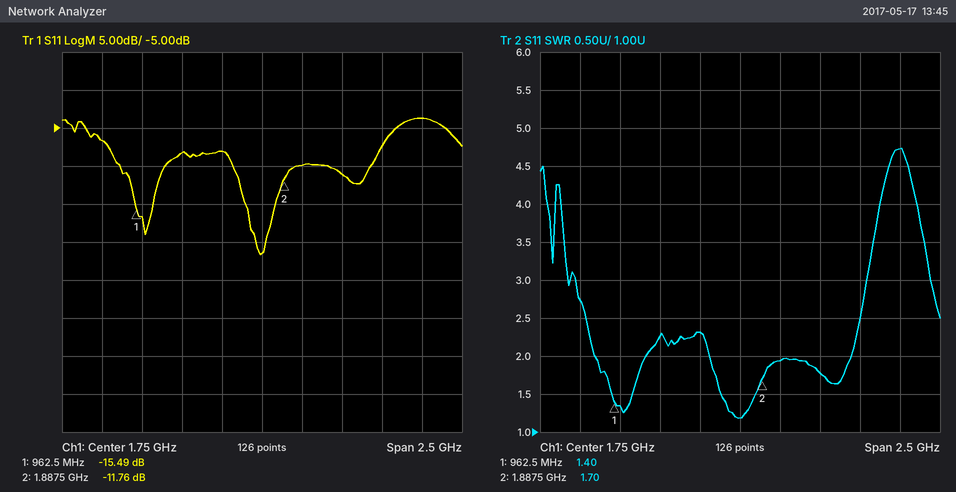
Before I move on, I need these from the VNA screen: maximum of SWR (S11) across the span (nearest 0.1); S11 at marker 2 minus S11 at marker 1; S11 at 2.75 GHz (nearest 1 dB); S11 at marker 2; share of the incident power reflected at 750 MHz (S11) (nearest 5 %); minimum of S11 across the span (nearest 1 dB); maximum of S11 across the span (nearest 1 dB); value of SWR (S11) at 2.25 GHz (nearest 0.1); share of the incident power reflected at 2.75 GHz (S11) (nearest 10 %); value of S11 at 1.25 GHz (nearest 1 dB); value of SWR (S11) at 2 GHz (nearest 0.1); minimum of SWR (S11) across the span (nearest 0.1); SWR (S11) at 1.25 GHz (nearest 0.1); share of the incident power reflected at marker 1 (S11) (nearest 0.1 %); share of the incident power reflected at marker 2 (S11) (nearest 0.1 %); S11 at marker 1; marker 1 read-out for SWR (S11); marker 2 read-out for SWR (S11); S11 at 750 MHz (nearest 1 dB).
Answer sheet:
4.7
3.73 dB
-4 dB
-11.76 dB
20 %
-22 dB
-4 dB
1.8
40 %
-8 dB
1.9
1.2
2.3
2.8 %
6.7 %
-15.49 dB
1.40
1.70
-7 dB
